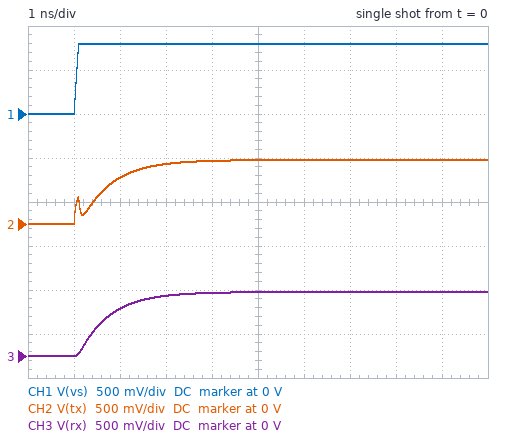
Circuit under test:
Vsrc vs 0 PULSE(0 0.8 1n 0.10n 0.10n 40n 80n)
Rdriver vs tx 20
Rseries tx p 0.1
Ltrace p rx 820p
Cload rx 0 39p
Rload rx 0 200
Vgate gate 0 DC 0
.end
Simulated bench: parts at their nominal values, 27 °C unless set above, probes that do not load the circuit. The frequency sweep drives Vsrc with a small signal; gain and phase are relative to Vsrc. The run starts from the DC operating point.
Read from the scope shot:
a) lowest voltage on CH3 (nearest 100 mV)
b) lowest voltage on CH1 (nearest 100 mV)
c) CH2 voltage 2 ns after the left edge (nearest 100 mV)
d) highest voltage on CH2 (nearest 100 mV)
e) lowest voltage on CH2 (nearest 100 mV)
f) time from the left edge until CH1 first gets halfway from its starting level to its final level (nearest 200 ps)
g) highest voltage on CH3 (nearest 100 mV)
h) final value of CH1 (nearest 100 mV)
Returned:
0 V
0 V
500 mV
700 mV
0 V
1.0 ns
700 mV
800 mV
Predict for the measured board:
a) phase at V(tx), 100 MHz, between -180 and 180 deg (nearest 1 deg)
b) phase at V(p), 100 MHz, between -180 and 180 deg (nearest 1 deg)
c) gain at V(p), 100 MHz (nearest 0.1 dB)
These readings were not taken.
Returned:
-24 deg
-24 deg
-1.7 dB
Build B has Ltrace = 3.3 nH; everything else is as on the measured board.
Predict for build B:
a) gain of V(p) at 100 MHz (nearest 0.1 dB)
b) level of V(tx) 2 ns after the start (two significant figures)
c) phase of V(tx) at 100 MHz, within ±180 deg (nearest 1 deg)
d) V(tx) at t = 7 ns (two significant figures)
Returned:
-1.8 dB
460 mV
-25 deg
730 mV
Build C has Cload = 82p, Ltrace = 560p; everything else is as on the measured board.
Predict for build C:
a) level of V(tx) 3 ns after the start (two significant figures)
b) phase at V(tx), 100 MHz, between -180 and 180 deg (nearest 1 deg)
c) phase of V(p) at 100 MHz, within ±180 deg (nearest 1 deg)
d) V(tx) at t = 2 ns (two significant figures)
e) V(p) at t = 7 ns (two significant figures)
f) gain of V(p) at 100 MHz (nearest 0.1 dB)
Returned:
530 mV
-43 deg
-44 deg
330 mV
710 mV
-3.7 dB
